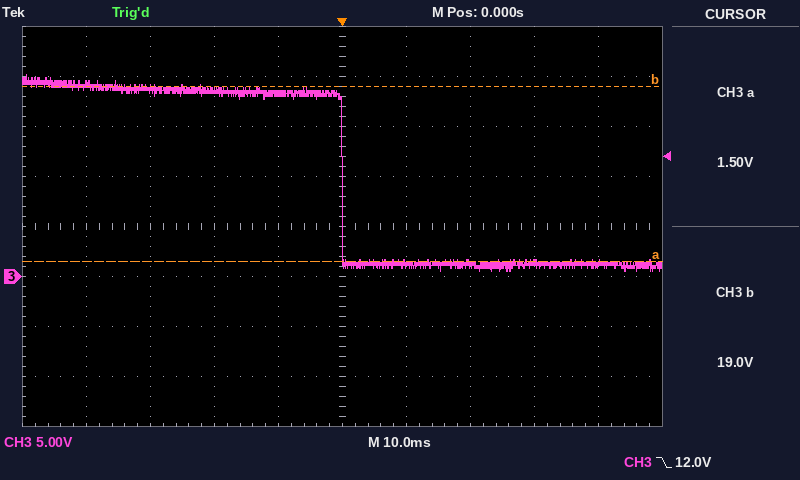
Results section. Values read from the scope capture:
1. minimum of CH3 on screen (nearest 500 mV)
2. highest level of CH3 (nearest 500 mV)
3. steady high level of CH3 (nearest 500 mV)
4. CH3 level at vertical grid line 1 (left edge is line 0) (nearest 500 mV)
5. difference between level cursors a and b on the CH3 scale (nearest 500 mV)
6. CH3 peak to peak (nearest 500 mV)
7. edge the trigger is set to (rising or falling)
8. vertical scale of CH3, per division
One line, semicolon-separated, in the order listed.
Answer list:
500 mV; 20.0 V; 18.5 V; 19.0 V; 17.5 V; 19.5 V; falling; 5 V
